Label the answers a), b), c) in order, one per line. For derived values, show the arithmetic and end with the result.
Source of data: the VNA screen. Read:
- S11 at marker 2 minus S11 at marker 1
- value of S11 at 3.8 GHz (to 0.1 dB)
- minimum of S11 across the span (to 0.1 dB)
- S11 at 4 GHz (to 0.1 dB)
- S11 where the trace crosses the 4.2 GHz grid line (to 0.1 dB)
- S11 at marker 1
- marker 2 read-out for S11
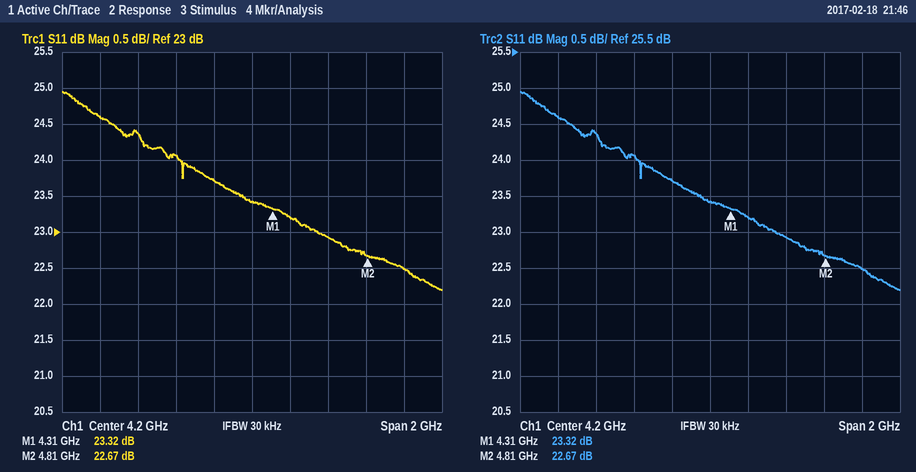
a) 22.67 − (23.32) = -0.65 dB
b) 24.1 dB
c) 22.2 dB
d) 23.7 dB
e) 23.4 dB
f) 23.32 dB
g) 22.67 dB
